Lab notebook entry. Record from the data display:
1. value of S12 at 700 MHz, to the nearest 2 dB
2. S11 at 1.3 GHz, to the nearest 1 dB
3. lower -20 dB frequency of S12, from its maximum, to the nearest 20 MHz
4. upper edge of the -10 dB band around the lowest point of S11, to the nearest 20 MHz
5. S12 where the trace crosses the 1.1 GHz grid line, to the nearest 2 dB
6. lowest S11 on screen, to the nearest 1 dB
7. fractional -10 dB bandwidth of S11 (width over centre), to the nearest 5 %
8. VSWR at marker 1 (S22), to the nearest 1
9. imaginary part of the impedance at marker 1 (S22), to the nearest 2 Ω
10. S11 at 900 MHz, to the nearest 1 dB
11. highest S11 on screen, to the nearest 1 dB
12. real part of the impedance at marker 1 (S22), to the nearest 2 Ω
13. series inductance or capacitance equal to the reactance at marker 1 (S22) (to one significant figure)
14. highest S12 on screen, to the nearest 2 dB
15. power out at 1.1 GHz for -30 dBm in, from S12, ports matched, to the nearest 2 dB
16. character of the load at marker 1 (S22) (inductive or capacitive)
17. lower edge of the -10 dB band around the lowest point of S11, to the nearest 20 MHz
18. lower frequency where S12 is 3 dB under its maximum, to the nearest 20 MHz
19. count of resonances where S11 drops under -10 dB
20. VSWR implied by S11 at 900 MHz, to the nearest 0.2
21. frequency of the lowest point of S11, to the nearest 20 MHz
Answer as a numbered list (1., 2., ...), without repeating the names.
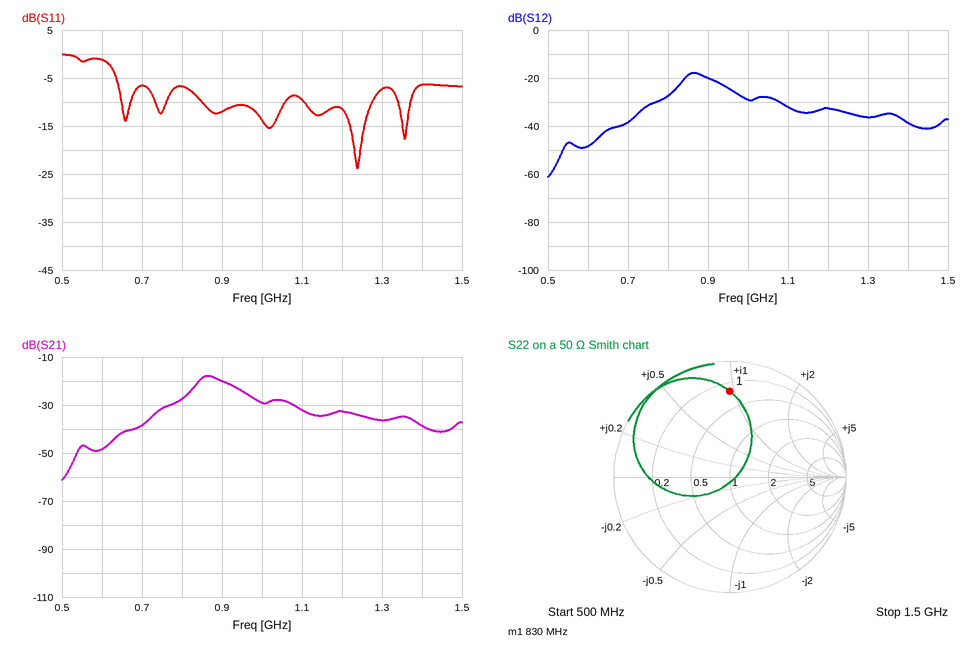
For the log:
1. -38 dB
2. -7 dB
3. 700 MHz
4. 1.28 GHz
5. -32 dB
6. -24 dB
7. 15 %
8. 7
9. +48 Ω
10. -12 dB
11. 0 dB
12. 14 Ω
13. 9 nH
14. -18 dB
15. -62 dBm
16. inductive
17. 1.10 GHz
18. 840 MHz
19. 5
20. 1.6
21. 1.24 GHz
